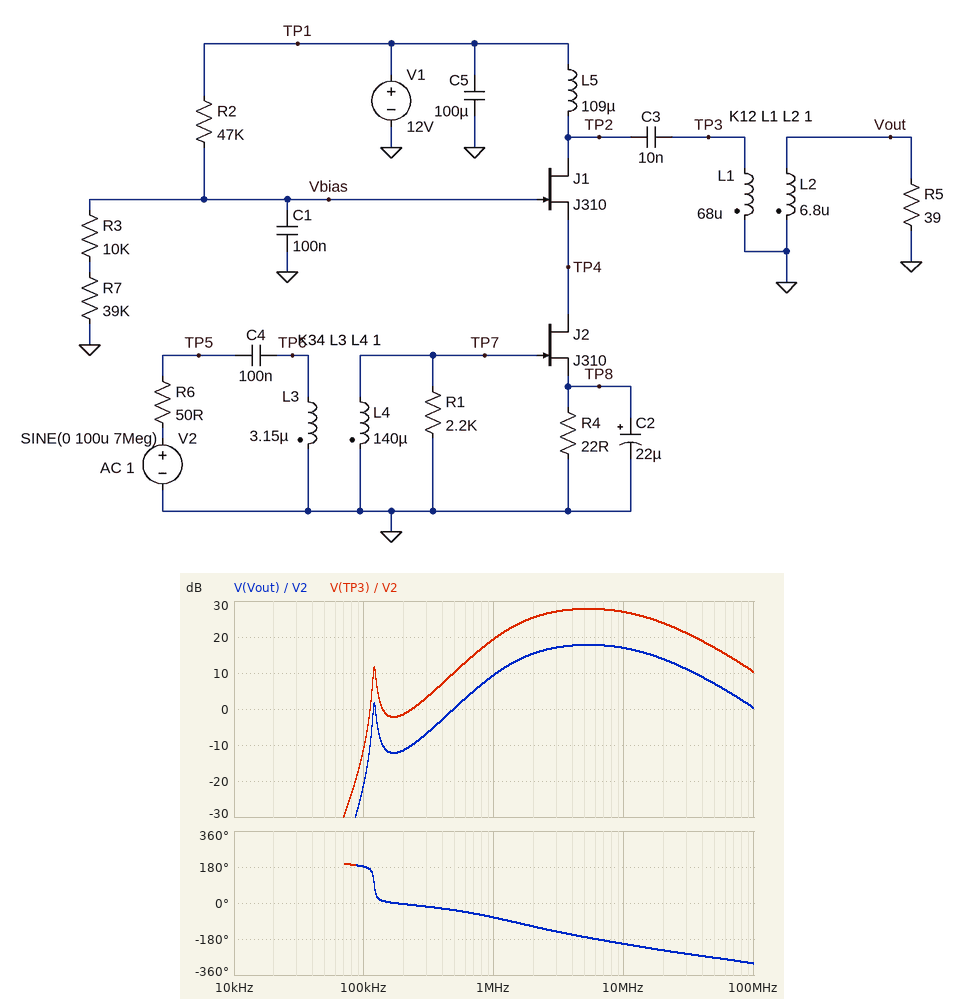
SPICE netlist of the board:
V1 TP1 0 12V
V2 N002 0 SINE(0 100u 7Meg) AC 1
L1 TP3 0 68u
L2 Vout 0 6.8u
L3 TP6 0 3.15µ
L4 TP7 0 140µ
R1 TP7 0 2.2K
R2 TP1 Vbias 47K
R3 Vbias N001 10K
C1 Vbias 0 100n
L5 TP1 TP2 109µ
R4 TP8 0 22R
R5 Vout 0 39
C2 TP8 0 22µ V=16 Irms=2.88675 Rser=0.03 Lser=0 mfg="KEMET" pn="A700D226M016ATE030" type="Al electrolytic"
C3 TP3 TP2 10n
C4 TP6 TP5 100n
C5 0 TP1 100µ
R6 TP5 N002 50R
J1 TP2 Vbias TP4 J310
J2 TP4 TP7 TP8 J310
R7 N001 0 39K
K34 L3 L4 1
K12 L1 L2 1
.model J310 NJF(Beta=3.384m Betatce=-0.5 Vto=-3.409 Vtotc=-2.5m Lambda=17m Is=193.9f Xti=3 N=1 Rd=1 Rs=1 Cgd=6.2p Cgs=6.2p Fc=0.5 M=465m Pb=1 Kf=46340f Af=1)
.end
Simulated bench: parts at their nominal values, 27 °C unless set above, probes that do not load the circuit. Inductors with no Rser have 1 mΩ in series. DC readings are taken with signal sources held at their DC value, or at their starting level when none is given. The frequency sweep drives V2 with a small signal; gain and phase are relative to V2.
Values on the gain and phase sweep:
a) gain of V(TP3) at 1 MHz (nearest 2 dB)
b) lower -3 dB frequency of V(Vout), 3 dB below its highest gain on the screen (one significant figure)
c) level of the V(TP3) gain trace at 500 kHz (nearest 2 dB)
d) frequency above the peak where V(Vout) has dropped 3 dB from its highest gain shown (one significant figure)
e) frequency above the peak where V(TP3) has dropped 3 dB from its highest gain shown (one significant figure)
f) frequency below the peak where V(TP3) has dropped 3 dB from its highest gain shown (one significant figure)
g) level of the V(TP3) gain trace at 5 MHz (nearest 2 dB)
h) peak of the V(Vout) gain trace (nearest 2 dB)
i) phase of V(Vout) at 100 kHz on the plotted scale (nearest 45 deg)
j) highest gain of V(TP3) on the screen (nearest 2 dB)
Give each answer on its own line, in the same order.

20 dB
2 MHz
10 dB
20 MHz
20 MHz
2 MHz
28 dB
18 dB
180 deg
28 dB
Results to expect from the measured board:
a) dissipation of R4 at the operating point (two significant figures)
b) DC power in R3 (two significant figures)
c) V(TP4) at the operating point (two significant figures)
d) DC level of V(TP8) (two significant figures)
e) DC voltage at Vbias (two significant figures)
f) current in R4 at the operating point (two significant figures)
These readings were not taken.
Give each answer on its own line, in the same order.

18 mW
160 µW
6.7 V
620 mV
6.1 V
28 mA
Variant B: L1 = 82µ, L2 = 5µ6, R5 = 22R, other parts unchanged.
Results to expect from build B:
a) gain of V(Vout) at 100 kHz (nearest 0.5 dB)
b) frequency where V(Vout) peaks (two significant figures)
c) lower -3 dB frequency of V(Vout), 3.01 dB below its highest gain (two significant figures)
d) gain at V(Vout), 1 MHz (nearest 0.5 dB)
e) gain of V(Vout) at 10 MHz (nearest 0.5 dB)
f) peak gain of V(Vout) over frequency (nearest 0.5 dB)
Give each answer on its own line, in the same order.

-19.0 dB
4.9 MHz
1.6 MHz
8.0 dB
13.5 dB
14.5 dB
